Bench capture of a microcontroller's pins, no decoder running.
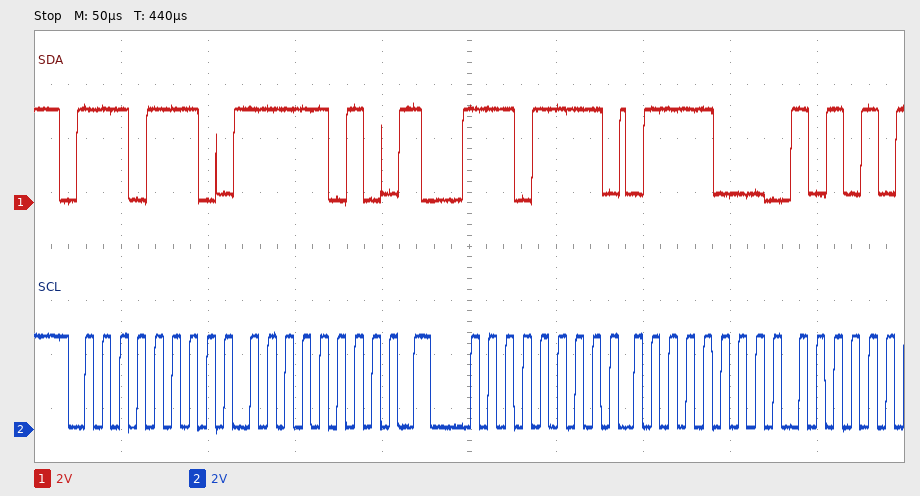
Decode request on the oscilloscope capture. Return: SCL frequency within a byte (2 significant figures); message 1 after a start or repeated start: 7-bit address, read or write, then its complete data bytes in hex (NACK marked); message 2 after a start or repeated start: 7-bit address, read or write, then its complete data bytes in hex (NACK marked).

100 kHz
0x77 write: FA
0x77 read: 78
